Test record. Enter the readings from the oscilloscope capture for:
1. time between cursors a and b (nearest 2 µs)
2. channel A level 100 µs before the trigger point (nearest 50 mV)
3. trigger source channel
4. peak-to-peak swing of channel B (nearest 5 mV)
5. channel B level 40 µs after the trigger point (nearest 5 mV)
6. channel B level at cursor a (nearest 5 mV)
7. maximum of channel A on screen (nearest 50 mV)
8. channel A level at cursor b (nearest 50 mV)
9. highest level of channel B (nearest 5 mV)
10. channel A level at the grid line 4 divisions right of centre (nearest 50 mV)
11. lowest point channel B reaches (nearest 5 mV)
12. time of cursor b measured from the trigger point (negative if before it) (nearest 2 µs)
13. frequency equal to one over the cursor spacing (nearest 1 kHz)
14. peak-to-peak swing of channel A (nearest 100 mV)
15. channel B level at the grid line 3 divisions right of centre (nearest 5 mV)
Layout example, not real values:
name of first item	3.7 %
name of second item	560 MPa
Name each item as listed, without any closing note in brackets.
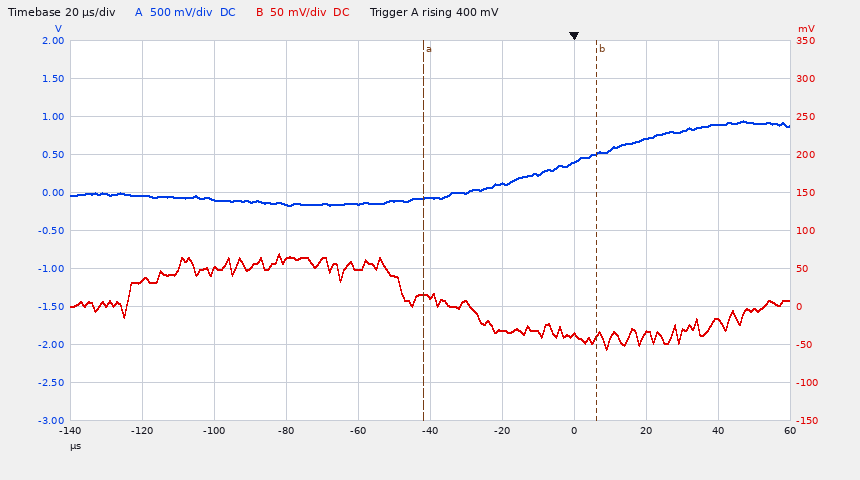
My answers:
time between cursors a and b	48 µs
channel A level 100 µs before the trigger point	-100 mV
trigger source channel	channel A
peak-to-peak swing of channel B	125 mV
channel B level 40 µs after the trigger point	-20 mV
channel B level at cursor a	15 mV
maximum of channel A on screen	950 mV
channel A level at cursor b	500 mV
highest level of channel B	70 mV
channel A level at the grid line 4 divisions right of centre	900 mV
lowest point channel B reaches	-55 mV
time of cursor b measured from the trigger point (negative if before it)	+6 µs
frequency equal to one over the cursor spacing	21 kHz
peak-to-peak swing of channel A	1.10 V
channel B level at the grid line 3 divisions right of centre	-35 mV
